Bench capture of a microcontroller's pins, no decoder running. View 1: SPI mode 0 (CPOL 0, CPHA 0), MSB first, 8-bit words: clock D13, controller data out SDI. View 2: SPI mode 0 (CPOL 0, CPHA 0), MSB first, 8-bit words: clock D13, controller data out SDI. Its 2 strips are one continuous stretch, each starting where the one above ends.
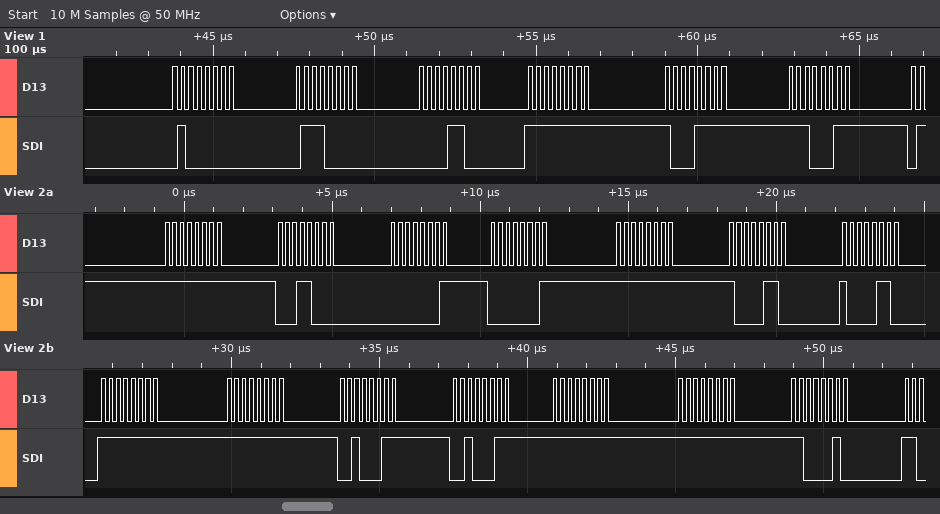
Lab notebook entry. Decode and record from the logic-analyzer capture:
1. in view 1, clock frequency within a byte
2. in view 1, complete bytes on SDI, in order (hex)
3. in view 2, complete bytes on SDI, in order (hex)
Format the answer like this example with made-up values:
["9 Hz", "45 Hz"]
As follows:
["4 MHz", "40 70 0C FF 8F E3", "FF 18 01 01 FF 86 86 FF FF 23 23 FF FF C2"]
